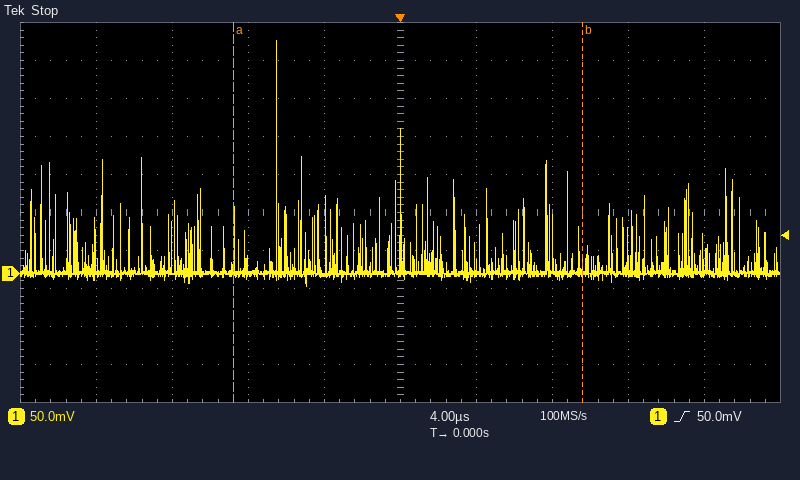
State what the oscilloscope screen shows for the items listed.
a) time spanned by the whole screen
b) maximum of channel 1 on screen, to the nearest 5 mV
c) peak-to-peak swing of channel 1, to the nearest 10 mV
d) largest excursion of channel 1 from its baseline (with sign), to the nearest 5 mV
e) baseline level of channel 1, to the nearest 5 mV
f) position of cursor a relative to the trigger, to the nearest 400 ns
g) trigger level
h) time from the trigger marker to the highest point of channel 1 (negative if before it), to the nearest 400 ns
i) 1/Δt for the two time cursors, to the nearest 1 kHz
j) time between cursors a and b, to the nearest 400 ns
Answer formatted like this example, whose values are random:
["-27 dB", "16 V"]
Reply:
["40 µs", "305 mV", "320 mV", "+305 mV", "0 mV", "-8.8 µs", "50.0 mV", "-6.4 µs", "54 kHz", "18.4 µs"]
